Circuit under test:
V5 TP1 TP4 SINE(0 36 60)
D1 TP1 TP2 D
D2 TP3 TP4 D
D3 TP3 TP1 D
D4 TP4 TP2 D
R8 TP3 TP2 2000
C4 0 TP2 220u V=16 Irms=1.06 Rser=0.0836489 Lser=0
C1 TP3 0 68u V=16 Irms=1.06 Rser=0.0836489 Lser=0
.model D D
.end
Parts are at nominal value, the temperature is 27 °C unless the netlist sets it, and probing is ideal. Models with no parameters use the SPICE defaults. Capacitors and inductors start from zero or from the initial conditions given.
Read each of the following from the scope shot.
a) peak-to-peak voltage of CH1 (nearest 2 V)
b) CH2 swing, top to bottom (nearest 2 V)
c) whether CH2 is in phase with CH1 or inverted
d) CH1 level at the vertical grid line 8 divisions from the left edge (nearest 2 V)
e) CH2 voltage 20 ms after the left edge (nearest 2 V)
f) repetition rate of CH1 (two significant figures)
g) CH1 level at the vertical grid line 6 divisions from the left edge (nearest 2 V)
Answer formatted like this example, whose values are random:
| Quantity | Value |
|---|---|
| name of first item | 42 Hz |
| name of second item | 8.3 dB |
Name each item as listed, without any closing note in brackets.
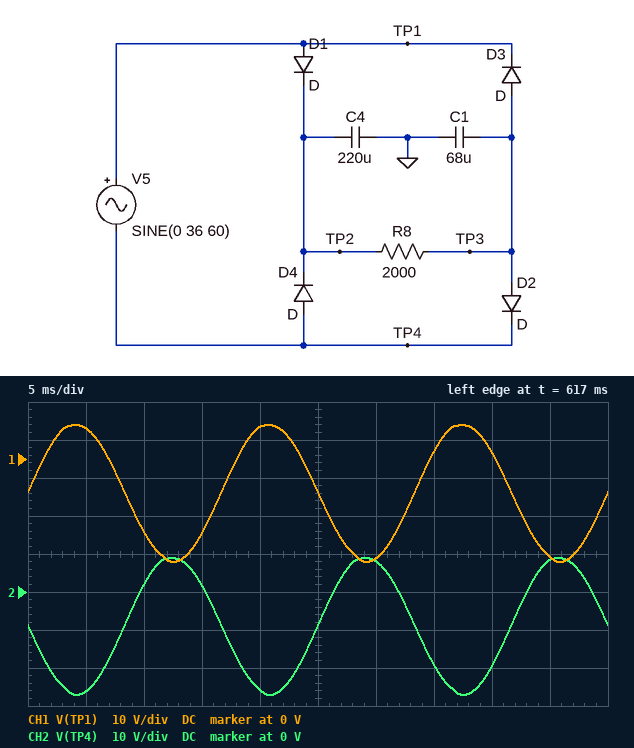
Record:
| Quantity | Value |
|---|---|
| peak-to-peak voltage of CH1 | 36 V |
| CH2 swing, top to bottom | 36 V |
| whether CH2 is in phase with CH1 or inverted | inverted |
| CH1 level at the vertical grid line 8 divisions from the left edge | 2 V |
| CH2 voltage 20 ms after the left edge | -26 V |
| repetition rate of CH1 | 60 Hz |
| CH1 level at the vertical grid line 6 divisions from the left edge | -26 V |
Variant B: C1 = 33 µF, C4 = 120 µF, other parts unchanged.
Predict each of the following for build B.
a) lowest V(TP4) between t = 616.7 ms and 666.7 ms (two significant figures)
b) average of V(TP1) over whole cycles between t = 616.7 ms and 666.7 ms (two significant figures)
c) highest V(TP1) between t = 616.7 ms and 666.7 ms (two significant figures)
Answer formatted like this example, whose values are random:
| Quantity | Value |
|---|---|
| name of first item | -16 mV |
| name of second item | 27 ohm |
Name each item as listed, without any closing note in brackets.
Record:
| Quantity | Value |
|---|---|
| lowest V(TP4) between t = 616.7 ms and 666.7 ms | -28 V |
| average of V(TP1) over whole cycles between t = 616.7 ms and 666.7 ms | -9.2 V |
| highest V(TP1) between t = 616.7 ms and 666.7 ms | 8.2 V |
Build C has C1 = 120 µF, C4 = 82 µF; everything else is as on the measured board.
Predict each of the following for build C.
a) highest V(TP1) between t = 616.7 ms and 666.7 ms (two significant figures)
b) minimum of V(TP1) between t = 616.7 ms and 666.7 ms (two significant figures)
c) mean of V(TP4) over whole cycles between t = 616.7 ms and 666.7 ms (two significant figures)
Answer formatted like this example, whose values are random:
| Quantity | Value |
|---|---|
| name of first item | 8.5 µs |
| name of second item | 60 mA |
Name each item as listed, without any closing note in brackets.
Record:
| Quantity | Value |
|---|---|
| highest V(TP1) between t = 616.7 ms and 666.7 ms | 21 V |
| minimum of V(TP1) between t = 616.7 ms and 666.7 ms | -15 V |
| mean of V(TP4) over whole cycles between t = 616.7 ms and 666.7 ms | 3.1 V |
